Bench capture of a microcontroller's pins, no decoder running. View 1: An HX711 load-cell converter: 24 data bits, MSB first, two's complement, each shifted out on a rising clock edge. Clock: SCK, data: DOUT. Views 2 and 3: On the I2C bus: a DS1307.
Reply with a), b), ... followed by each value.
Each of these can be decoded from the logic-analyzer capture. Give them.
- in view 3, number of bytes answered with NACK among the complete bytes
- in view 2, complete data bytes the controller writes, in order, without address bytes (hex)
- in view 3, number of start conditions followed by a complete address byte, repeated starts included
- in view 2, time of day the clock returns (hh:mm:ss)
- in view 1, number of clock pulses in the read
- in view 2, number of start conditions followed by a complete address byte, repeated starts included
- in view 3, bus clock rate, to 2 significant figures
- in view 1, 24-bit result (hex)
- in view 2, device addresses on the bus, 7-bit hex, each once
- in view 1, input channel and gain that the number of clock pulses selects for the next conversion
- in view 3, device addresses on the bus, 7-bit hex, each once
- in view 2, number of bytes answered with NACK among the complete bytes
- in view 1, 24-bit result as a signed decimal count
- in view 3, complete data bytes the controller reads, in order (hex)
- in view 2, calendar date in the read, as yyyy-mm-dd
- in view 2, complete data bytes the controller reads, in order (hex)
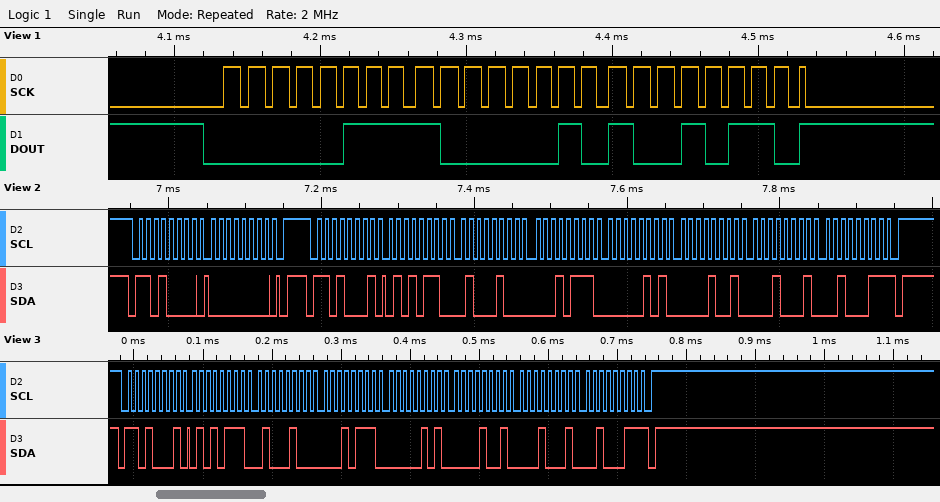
a) 1
b) 00
c) 1
d) 17:44:56
e) 25
f) 2
g) 100 kHz
h) 0x078296
i) 0x68
j) channel A, gain 128
k) 0x68
l) 1
m) 492182
n) 57 44 17 05 09 11 23
o) 2023-11-09
p) 56 44 17 05 09 11 23
